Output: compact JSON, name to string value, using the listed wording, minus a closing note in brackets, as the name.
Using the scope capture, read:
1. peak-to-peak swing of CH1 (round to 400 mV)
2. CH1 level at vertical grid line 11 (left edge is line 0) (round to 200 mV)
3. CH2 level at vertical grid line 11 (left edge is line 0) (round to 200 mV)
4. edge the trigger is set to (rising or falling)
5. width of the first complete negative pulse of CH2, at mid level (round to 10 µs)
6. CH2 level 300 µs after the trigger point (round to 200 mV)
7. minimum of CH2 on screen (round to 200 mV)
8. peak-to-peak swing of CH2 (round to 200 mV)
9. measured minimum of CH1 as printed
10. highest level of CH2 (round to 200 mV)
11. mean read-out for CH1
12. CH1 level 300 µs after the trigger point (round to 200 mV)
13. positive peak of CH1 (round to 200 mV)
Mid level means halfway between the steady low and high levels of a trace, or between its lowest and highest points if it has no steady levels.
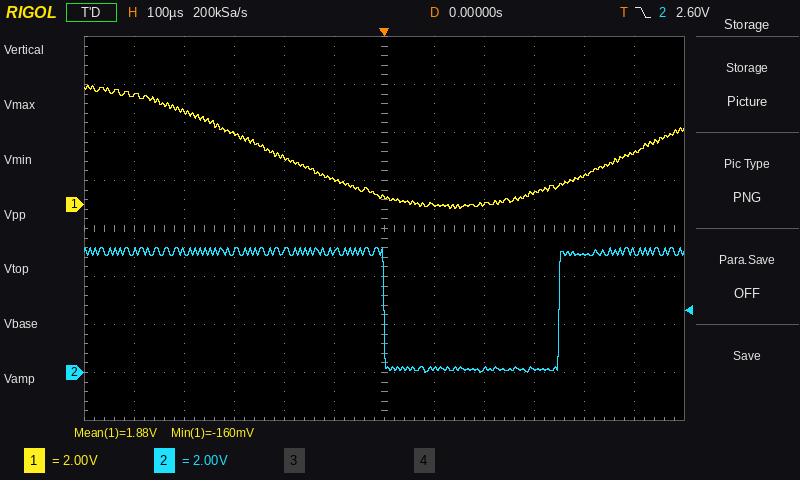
{"peak-to-peak swing of CH1": "5.2 V", "CH1 level at vertical grid line 11 (left edge is line 0)": "2.2 V", "CH2 level at vertical grid line 11 (left edge is line 0)": "5.0 V", "edge the trigger is set to": "falling", "width of the first complete negative pulse of CH2, at mid level": "350 µs", "CH2 level 300 µs after the trigger point": "200 mV", "minimum of CH2 on screen": "0.0 V", "peak-to-peak swing of CH2": "5.2 V", "measured minimum of CH1 as printed": "-160 mV", "highest level of CH2": "5.2 V", "mean read-out for CH1": "1.88 V", "CH1 level 300 µs after the trigger point": "400 mV", "positive peak of CH1": "5.0 V"}
